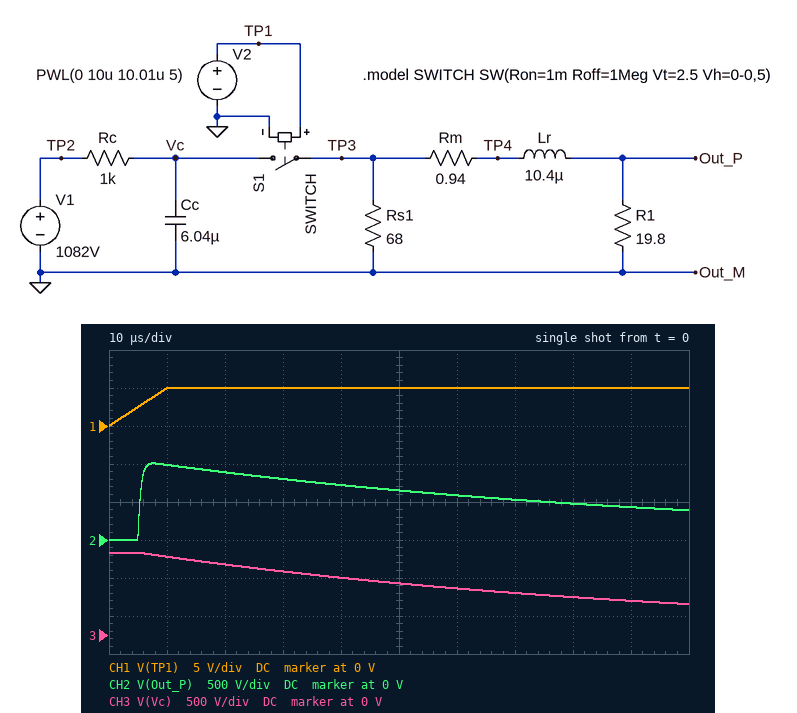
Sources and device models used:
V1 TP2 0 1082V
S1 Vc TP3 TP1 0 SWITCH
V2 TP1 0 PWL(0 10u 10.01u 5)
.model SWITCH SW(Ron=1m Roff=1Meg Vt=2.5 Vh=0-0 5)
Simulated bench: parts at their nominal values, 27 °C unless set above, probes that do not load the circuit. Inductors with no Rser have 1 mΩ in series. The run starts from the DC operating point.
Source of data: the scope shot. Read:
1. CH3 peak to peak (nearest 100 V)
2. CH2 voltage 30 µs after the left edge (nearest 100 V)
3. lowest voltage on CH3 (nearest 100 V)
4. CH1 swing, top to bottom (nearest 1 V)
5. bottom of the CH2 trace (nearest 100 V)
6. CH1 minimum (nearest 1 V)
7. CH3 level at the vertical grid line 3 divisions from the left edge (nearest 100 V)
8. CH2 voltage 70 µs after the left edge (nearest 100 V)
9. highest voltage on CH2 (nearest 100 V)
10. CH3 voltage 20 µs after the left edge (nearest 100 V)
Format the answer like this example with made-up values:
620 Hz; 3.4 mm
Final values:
700 V; 800 V; 400 V; 5 V; 0 V; 0 V; 800 V; 500 V; 1.0 kV; 900 V
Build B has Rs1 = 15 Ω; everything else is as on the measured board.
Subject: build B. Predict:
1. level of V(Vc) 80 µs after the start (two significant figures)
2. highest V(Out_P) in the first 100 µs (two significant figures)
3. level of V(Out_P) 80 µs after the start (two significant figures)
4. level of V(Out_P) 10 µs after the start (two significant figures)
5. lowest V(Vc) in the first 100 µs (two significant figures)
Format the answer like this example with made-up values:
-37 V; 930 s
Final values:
260 V; 990 V; 250 V; 950 V; 180 V
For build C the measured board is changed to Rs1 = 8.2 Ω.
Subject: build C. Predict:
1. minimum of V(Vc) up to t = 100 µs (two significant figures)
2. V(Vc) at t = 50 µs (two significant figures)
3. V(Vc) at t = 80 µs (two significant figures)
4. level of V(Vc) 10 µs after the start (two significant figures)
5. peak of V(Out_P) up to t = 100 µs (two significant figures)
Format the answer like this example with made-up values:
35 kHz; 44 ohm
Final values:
79 V; 310 V; 130 V; 940 V; 970 V
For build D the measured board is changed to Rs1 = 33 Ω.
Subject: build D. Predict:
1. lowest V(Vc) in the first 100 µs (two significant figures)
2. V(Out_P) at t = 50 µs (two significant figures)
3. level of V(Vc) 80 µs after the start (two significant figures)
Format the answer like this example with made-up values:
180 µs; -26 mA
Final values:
320 V; 580 V; 410 V
